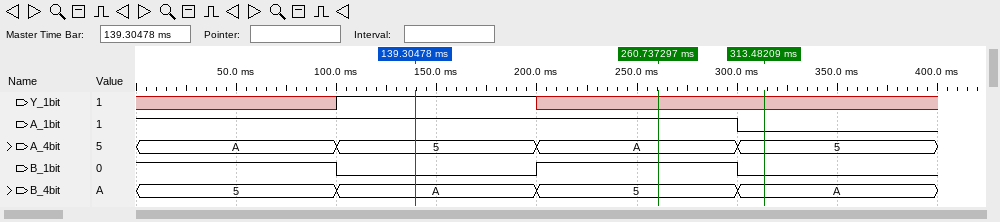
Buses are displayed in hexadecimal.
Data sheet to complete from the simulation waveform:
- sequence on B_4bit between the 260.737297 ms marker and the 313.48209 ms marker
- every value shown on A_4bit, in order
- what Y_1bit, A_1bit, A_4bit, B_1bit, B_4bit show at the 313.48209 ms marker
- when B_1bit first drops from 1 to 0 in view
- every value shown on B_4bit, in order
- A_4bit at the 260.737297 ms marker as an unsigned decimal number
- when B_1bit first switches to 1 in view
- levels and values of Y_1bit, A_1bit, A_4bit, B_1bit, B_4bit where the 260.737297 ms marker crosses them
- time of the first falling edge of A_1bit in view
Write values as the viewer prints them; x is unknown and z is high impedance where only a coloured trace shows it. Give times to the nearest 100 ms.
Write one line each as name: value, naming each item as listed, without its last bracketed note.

sequence on B_4bit between the 260.737297 ms marker and the 313.48209 ms marker: 5, A
every value shown on A_4bit, in order: A, 5, A, 5
what Y_1bit, A_1bit, A_4bit, B_1bit, B_4bit show at the 313.48209 ms marker: Y_1bit=x, A_1bit=0, A_4bit=5, B_1bit=0, B_4bit=A
when B_1bit first drops from 1 to 0 in view: 100 ms
every value shown on B_4bit, in order: 5, A, 5, A
A_4bit at the 260.737297 ms marker as an unsigned decimal number: 10
when B_1bit first switches to 1 in view: 200 ms
levels and values of Y_1bit, A_1bit, A_4bit, B_1bit, B_4bit where the 260.737297 ms marker crosses them: Y_1bit=x, A_1bit=1, A_4bit=A, B_1bit=1, B_4bit=5
time of the first falling edge of A_1bit in view: 300 ms
